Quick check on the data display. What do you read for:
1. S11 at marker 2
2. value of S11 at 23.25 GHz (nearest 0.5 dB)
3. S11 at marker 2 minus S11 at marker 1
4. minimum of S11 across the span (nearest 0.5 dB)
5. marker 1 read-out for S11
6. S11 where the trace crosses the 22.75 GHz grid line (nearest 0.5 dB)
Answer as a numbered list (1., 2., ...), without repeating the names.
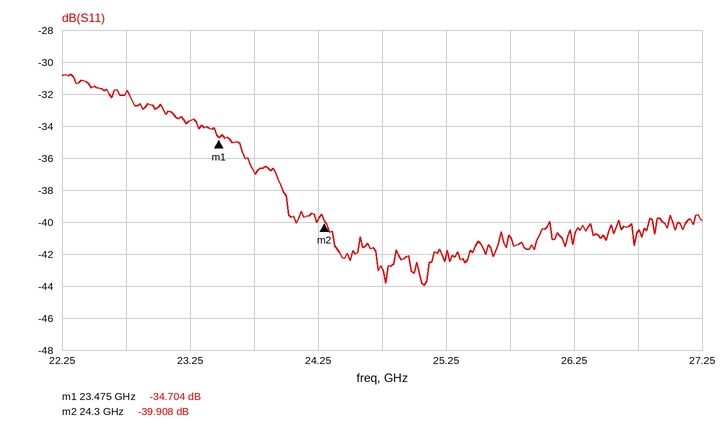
1. -39.908 dB
2. -33.5 dB
3. -5.204 dB
4. -44.0 dB
5. -34.704 dB
6. -32.0 dB
